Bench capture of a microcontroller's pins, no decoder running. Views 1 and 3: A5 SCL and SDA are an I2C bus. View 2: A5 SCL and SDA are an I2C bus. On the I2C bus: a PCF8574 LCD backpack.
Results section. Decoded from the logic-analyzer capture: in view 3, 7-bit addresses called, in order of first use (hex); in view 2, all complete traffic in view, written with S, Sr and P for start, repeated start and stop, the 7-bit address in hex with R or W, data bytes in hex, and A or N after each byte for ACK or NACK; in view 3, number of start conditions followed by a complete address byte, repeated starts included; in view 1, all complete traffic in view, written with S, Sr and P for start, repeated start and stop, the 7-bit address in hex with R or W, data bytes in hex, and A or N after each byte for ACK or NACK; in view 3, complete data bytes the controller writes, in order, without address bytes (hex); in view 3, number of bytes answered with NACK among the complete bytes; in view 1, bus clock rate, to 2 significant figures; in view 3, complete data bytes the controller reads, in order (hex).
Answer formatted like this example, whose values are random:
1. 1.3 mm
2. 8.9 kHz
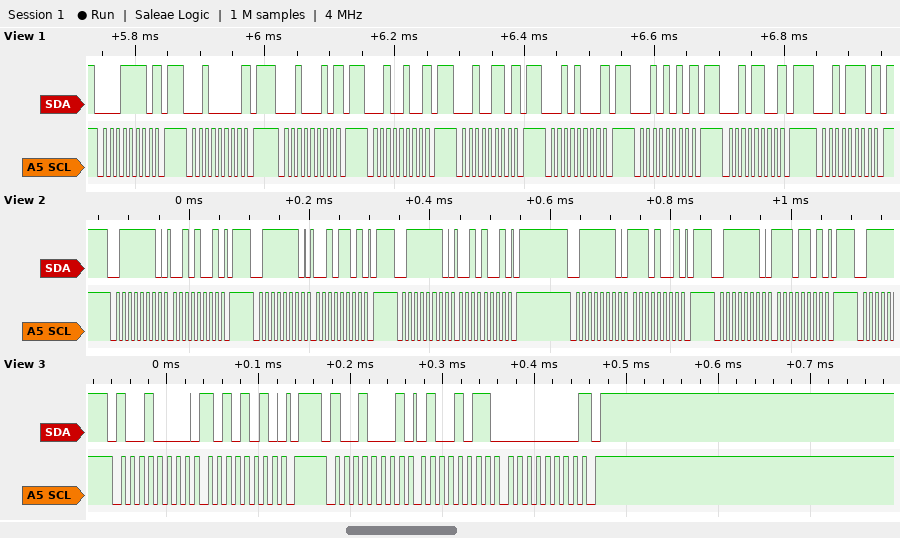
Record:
1. 0x48
2. S 3FW A 29 A P S 3FW A 2D A P S 3FW A 29 A P S 3FW A E9 A P S 3FW A ED A P
3. 2
4. S 0FW N P S 10W N P S 11W N P S 12W N P S 13W N P S 14W N P S 15W N P S 16W N P S 17W N P
5. AA
6. 1
7. 100 kHz
8. 4B 00
